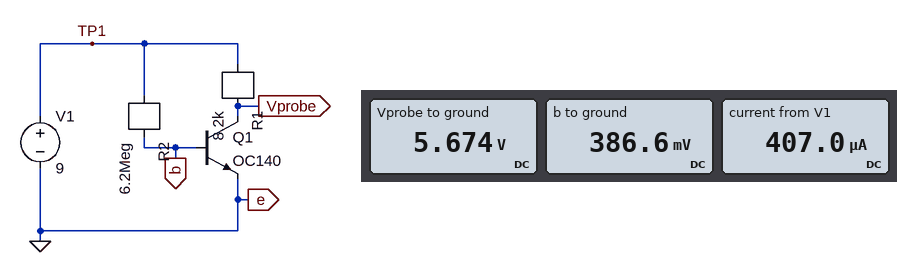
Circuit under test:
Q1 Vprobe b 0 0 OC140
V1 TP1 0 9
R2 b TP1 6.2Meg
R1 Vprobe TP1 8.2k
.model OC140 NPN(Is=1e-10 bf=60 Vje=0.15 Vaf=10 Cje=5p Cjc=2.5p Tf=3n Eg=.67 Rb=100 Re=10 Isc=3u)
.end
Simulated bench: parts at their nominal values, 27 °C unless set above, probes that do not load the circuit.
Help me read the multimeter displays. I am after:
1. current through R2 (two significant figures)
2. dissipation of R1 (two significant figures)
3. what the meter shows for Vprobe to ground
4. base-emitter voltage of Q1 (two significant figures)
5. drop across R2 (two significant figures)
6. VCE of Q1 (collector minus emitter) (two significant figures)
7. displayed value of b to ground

1.4 µA
1.3 mW
5.674 V
390 mV
8.6 V
5.7 V
386.6 mV
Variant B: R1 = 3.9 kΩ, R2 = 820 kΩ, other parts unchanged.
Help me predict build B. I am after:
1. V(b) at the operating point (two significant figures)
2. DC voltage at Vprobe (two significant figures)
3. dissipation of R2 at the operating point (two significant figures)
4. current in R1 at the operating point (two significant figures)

420 mV
4.5 V
90 µW
1.1 mA
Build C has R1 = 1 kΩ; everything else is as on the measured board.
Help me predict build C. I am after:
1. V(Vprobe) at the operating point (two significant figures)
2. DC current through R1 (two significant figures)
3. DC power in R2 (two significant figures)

8.5 V
480 µA
12 µW
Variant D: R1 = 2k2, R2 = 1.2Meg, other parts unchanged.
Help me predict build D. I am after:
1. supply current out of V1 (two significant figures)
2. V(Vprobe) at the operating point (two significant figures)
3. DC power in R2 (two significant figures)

1.0 mA
6.8 V
61 µW
